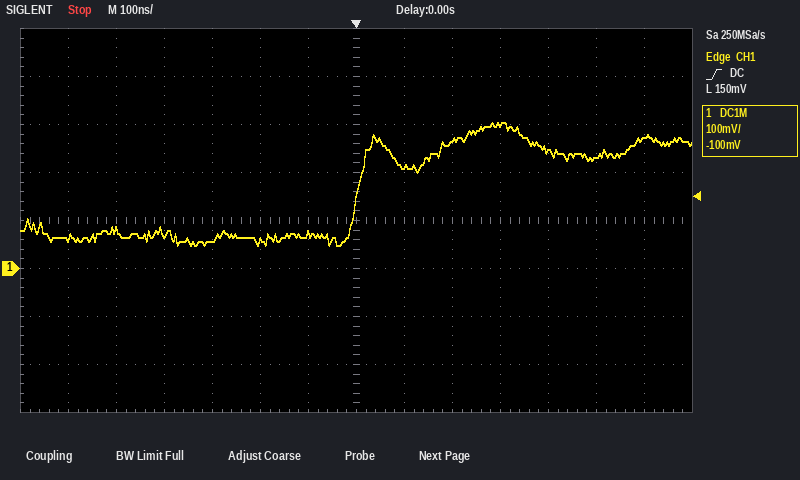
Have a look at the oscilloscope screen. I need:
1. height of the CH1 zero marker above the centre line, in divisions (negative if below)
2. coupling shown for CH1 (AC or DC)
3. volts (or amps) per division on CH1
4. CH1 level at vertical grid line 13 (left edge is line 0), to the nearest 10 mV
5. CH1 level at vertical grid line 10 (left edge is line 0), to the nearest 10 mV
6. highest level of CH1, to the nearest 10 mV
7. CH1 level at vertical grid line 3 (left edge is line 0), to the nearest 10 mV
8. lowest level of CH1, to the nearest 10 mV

-1.0 div
DC
100 mV
270 mV
300 mV
300 mV
70 mV
50 mV
